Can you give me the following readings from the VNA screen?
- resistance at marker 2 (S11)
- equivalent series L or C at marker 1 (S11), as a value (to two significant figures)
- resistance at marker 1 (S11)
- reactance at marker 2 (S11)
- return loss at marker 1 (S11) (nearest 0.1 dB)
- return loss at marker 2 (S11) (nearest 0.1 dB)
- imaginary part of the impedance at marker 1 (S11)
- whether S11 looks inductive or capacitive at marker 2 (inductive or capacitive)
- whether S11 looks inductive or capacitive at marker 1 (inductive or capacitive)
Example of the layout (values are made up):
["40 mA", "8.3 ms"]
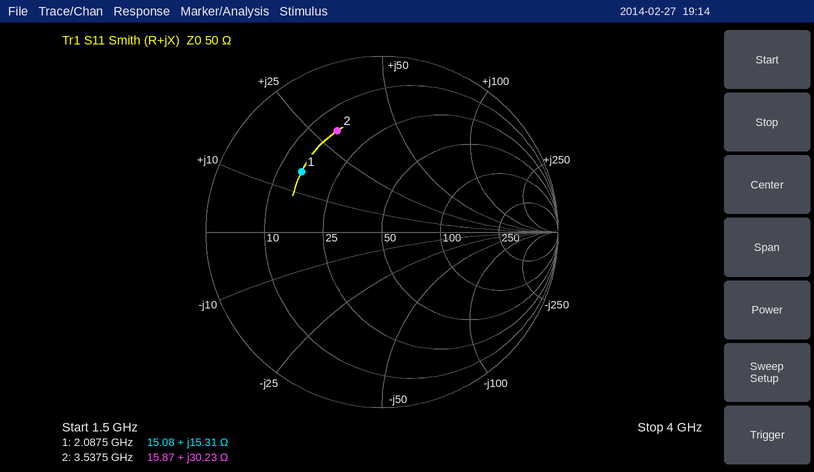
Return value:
["15.87 Ω", "1.2 nH", "15.08 Ω", "+30.23 Ω", "4.9 dB", "4.0 dB", "+15.31 Ω", "inductive", "inductive"]
